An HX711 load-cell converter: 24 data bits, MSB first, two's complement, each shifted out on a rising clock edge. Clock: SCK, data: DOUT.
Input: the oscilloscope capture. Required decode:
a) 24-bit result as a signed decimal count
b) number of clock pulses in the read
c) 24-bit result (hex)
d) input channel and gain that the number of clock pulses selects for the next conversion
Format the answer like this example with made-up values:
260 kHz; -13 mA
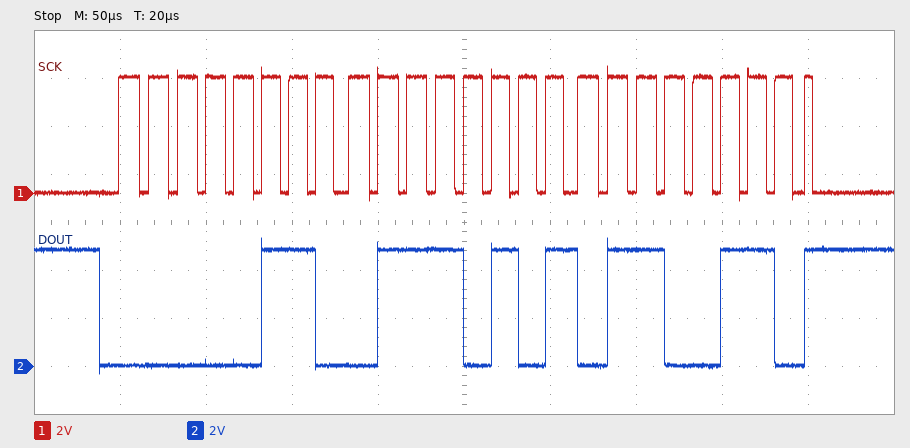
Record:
423270; 25; 0x067566; channel A, gain 128
